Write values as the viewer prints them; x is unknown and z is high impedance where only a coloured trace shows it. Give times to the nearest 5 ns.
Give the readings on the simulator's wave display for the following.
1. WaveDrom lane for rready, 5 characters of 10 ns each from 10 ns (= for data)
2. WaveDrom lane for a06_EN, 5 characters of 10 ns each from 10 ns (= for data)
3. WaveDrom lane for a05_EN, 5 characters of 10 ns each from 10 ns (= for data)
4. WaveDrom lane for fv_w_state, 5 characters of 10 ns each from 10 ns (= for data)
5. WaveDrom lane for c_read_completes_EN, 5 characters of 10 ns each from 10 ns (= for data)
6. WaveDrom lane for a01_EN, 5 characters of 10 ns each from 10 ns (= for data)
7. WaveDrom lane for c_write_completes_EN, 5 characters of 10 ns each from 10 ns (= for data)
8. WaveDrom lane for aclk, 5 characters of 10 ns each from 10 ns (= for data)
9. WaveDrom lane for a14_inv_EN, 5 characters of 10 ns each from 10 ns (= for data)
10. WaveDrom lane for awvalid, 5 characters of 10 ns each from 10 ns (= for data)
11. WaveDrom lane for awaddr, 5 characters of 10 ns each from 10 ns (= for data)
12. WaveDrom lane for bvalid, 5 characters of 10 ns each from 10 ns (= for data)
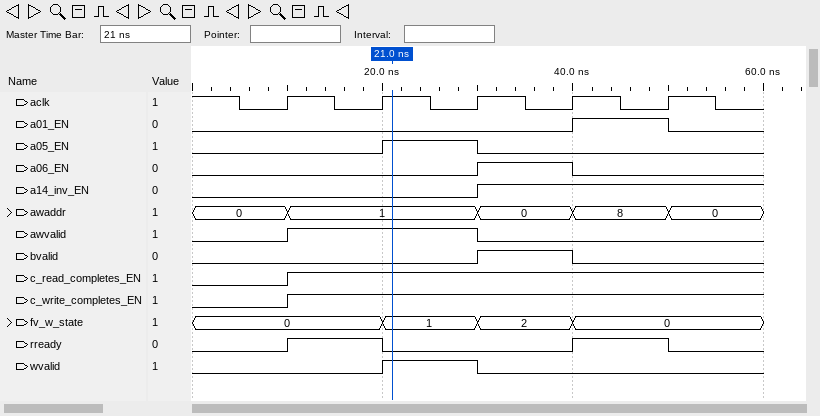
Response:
{name: 'rready', wave: '10.10'}
{name: 'a06_EN', wave: '0.10.'}
{name: 'a05_EN', wave: '010..'}
{name: 'fv_w_state', wave: '====.', data: '0 1 2 0'}
{name: 'c_read_completes_EN', wave: '1....'}
{name: 'a01_EN', wave: '0..10'}
{name: 'c_write_completes_EN', wave: '1....'}
{name: 'aclk', wave: 'p....'}
{name: 'a14_inv_EN', wave: '0.1..'}
{name: 'awvalid', wave: '1.0..'}
{name: 'awaddr', wave: '=.===', data: '1 0 8 0'}
{name: 'bvalid', wave: '0.10.'}
